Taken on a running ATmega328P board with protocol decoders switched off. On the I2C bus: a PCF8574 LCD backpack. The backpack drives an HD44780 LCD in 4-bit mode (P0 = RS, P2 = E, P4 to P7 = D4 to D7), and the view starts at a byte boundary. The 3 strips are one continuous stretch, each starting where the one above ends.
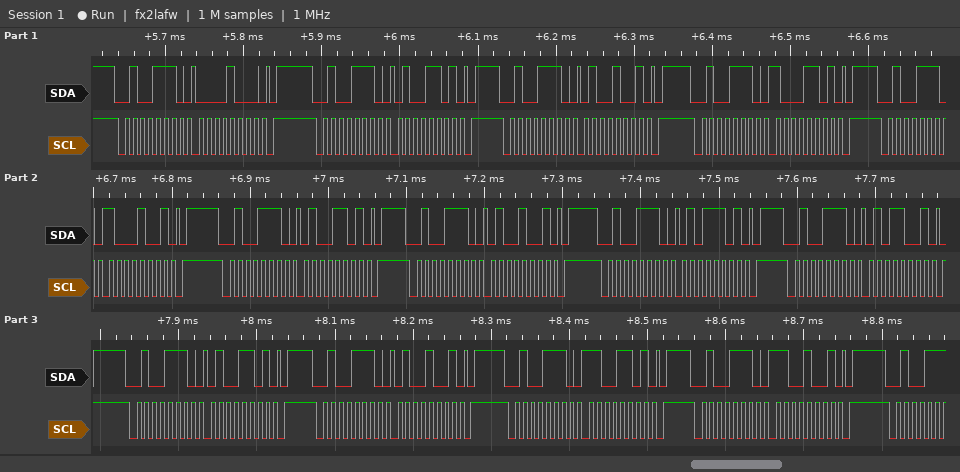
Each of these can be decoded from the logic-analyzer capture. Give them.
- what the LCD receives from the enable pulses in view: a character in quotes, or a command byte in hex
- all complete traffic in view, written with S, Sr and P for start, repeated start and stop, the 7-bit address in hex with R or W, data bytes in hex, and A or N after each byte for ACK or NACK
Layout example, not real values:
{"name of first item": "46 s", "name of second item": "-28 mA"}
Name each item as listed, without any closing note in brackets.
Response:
{"what the LCD receives from the enable pulses in view: a character in quotes, or a command byte in hex": "'H' 'E' 'L'", "all complete traffic in view, written with S, Sr and P for start, repeated start and stop, the 7-bit address in hex with R or W, data bytes in hex, and A or N after each byte for ACK or NACK": "S 27W A 08 A P S 27W A 4D A P S 27W A 49 A P S 27W A 8D A P S 27W A 89 A P S 27W A 4D A P S 27W A 49 A P S 27W A 5D A P S 27W A 59 A P S 27W A 4D A P S 27W A 49 A P S 27W A CD A P S 27W A C9 A P"}
